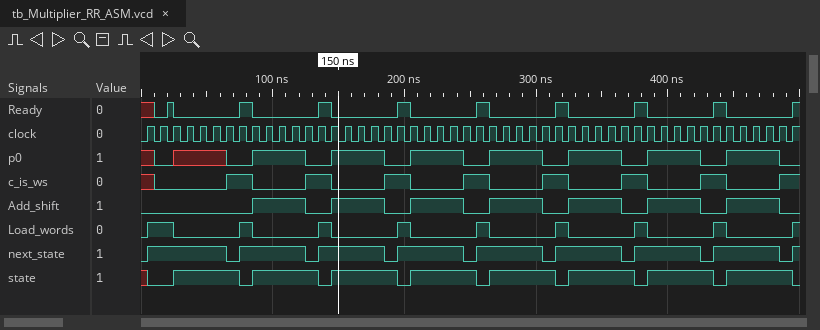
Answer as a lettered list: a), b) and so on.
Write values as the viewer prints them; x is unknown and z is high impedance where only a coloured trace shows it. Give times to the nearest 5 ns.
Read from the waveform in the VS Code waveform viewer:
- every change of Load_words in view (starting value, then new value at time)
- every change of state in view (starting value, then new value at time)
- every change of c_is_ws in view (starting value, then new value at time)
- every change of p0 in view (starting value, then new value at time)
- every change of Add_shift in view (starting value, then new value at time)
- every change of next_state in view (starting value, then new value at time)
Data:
a) 0, 1 at 5 ns, 0 at 25 ns, 1 at 75 ns, 0 at 85 ns, 1 at 135 ns, 0 at 145 ns, 1 at 195 ns, 0 at 205 ns, 1 at 255 ns, 0 at 265 ns, 1 at 315 ns, 0 at 325 ns, 1 at 375 ns, 0 at 385 ns, 1 at 435 ns, 0 at 445 ns, 1 at 495 ns
b) x, 0 at 5 ns, 1 at 25 ns, 0 at 75 ns, 1 at 85 ns, 0 at 135 ns, 1 at 145 ns, 0 at 195 ns, 1 at 205 ns, 0 at 255 ns, 1 at 265 ns, 0 at 315 ns, 1 at 325 ns, 0 at 375 ns, 1 at 385 ns, 0 at 435 ns, 1 at 445 ns, 0 at 495 ns
c) x, 0 at 10 ns, 1 at 65 ns, 0 at 85 ns, 1 at 125 ns, 0 at 145 ns, 1 at 185 ns, 0 at 205 ns, 1 at 245 ns, 0 at 265 ns, 1 at 305 ns, 0 at 325 ns, 1 at 365 ns, 0 at 385 ns, 1 at 425 ns, 0 at 445 ns, 1 at 485 ns
d) x, 0 at 10 ns, x at 25 ns, 0 at 65 ns, 1 at 85 ns, 0 at 125 ns, 1 at 145 ns, 0 at 185 ns, 1 at 205 ns, 0 at 245 ns, 1 at 265 ns, 0 at 305 ns, 1 at 325 ns, 0 at 365 ns, 1 at 385 ns, 0 at 425 ns, 1 at 445 ns, 0 at 485 ns
e) 0, 1 at 85 ns, 0 at 125 ns, 1 at 145 ns, 0 at 185 ns, 1 at 205 ns, 0 at 245 ns, 1 at 265 ns, 0 at 305 ns, 1 at 325 ns, 0 at 365 ns, 1 at 385 ns, 0 at 425 ns, 1 at 445 ns, 0 at 485 ns
f) 0, 1 at 5 ns, 0 at 65 ns, 1 at 75 ns, 0 at 125 ns, 1 at 135 ns, 0 at 185 ns, 1 at 195 ns, 0 at 245 ns, 1 at 255 ns, 0 at 305 ns, 1 at 315 ns, 0 at 365 ns, 1 at 375 ns, 0 at 425 ns, 1 at 435 ns, 0 at 485 ns, 1 at 495 ns
